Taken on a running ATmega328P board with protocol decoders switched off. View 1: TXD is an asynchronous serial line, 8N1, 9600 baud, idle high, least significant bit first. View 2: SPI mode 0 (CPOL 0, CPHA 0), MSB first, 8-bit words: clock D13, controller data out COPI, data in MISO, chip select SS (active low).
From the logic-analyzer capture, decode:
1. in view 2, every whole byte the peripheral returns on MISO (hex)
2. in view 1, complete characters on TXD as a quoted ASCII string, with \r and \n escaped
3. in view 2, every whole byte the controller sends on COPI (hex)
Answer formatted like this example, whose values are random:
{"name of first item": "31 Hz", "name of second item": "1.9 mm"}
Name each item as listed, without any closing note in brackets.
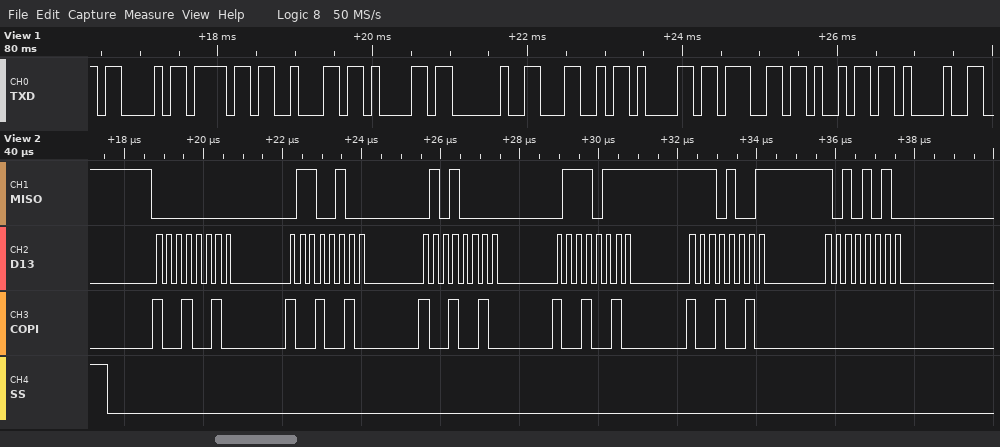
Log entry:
{"in view 2, every whole byte the peripheral returns on MISO": "00 64 50 77 E9 AA", "in view 1, complete characters on TXD as a quoted ASCII string, with \\r and \\n escaped": "\"Coba Lagi!\"", "in view 2, every whole byte the controller sends on COPI": "92 92 92 92 92 00"}
